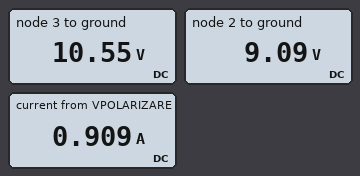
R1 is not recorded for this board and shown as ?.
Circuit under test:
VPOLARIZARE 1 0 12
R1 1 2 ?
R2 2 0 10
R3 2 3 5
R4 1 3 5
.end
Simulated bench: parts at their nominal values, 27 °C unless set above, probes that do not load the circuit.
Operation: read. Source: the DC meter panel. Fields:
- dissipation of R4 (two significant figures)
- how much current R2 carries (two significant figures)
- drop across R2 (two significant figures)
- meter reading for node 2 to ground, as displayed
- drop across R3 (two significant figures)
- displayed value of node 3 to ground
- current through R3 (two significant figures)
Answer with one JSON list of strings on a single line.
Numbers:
["420 mW", "910 mA", "9.1 V", "9.09 V", "1.5 V", "10.55 V", "290 mA"]
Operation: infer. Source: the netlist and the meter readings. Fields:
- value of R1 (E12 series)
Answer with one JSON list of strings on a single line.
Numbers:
["4.7 Ω"]
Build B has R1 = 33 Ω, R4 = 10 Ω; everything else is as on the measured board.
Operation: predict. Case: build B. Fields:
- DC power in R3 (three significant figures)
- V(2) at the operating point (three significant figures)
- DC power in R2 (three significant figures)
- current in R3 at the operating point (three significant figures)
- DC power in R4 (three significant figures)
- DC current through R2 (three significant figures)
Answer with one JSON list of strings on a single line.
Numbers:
["825 mW", "5.91 V", "3.49 W", "406 mA", "1.65 W", "591 mA"]
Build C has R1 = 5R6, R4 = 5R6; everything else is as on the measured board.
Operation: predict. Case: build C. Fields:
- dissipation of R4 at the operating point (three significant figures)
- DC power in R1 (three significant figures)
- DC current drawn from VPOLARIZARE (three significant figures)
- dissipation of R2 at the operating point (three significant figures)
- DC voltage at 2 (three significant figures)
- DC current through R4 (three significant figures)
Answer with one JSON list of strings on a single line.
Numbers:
["516 mW", "1.85 W", "878 mA", "7.71 W", "8.78 V", "304 mA"]
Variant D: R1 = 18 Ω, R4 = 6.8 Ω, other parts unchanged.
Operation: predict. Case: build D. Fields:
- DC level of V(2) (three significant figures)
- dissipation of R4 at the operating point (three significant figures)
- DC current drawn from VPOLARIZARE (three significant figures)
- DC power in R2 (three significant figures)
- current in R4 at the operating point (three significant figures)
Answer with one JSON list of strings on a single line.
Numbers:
["7.01 V", "1.22 W", "701 mA", "4.91 W", "423 mA"]
